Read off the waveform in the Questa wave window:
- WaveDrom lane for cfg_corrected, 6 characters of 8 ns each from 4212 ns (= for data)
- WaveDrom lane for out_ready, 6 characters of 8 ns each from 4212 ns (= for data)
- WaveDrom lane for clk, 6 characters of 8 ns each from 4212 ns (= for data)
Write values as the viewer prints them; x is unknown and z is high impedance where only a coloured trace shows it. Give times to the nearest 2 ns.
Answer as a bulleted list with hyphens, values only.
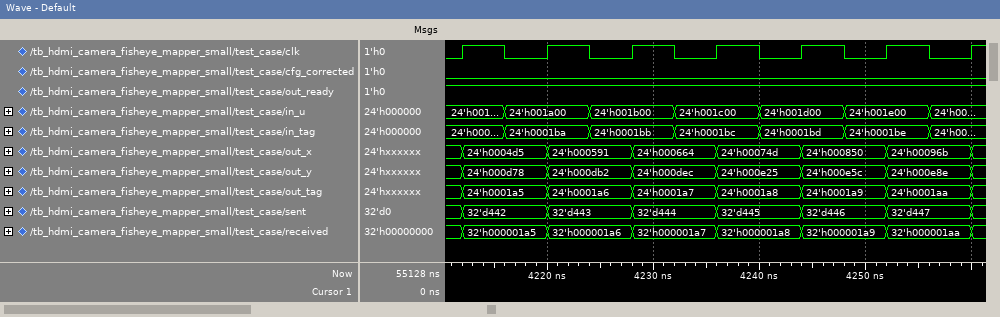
- {name: 'cfg_corrected', wave: '0.....'}
- {name: 'out_ready', wave: '1.....'}
- {name: 'clk', wave: 'p.....'}
